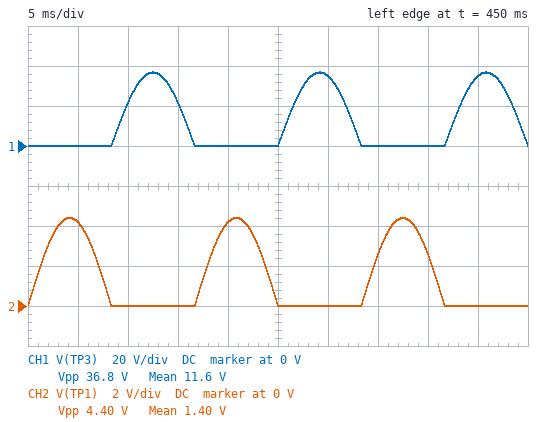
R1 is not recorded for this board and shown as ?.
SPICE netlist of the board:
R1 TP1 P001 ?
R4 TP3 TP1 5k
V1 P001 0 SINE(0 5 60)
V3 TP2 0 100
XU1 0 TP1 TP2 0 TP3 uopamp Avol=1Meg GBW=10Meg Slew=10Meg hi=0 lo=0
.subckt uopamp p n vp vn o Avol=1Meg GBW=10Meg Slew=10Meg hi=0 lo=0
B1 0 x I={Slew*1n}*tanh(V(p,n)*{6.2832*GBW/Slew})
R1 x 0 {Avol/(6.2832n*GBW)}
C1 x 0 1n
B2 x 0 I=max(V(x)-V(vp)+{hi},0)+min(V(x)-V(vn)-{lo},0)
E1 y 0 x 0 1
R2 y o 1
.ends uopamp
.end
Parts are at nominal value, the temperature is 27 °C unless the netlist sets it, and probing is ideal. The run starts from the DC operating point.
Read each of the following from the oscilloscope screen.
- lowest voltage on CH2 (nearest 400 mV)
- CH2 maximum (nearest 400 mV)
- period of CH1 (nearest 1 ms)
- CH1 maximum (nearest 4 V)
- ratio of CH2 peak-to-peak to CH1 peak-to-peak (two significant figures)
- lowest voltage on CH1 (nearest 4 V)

0 V
4.4 V
17 ms
36 V
0.12
0 V
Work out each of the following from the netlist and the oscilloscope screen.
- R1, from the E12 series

680 Ω
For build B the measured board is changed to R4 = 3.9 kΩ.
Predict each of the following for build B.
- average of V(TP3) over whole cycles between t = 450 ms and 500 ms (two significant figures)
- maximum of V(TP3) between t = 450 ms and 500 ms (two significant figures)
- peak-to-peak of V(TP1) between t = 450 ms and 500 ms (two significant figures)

9.1 V
29 V
4.3 V
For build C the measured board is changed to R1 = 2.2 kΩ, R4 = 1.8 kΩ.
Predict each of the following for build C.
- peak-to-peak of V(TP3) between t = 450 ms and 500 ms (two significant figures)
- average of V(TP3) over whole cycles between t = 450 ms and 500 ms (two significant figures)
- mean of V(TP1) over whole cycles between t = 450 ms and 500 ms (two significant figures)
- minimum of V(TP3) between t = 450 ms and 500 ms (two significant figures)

4.1 V
1.3 V
710 mV
-9.7 mV
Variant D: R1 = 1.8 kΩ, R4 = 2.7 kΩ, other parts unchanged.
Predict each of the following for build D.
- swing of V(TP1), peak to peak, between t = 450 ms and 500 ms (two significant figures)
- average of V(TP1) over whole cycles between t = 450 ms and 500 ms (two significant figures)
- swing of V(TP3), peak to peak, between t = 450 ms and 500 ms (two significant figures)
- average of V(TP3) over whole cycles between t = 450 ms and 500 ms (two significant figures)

3.0 V
950 mV
7.5 V
2.4 V
